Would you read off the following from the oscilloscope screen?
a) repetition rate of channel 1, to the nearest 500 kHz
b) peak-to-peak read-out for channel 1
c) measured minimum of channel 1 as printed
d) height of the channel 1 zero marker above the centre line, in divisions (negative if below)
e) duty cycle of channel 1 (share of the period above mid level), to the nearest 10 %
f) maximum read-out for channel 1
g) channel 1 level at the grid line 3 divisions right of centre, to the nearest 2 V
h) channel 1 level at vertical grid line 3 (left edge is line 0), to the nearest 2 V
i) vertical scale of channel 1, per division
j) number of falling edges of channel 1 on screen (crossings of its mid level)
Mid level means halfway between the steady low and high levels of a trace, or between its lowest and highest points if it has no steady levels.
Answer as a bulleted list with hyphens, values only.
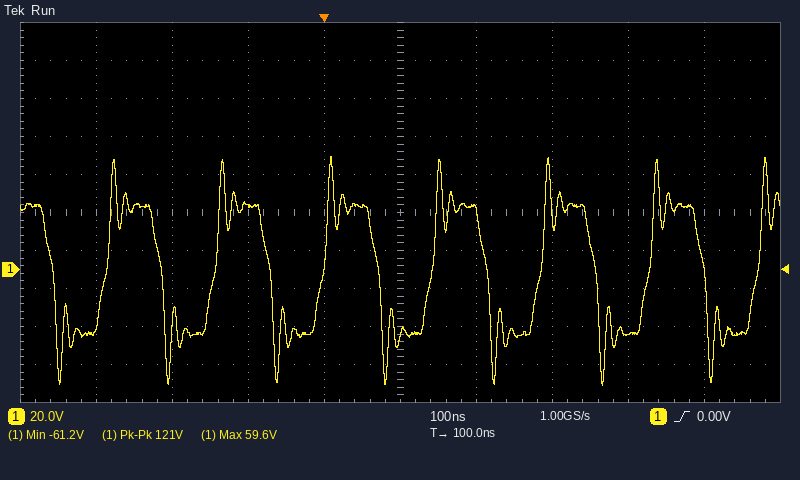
- 7.0 MHz
- 121 V
- -61.2 V
- -1.5 div
- 50 %
- 59.6 V
- -34 V
- 34 V
- 20 V
- 7
